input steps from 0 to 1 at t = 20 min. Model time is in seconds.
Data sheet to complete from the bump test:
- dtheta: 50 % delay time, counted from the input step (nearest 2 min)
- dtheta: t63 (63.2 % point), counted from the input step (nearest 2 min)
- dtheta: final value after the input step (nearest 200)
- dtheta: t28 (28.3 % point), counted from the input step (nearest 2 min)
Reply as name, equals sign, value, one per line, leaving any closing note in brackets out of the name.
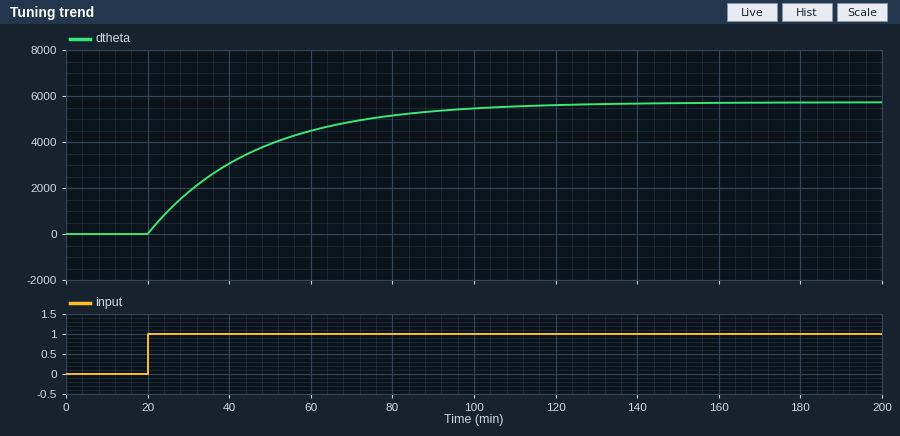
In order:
dtheta: 50 % delay time, counted from the input step = 18 min
dtheta: t63 (63.2 % point), counted from the input step = 26 min
dtheta: final value after the input step = 5800
dtheta: t28 (28.3 % point), counted from the input step = 8 min
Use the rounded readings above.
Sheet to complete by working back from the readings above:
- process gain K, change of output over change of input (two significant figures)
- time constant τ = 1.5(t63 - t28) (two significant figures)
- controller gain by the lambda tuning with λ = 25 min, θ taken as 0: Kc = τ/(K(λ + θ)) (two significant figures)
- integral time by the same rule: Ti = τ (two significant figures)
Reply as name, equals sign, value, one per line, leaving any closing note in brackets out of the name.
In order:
process gain K, change of output over change of input = 5800
time constant τ = 1.5(t63 - t28) = 27 min
controller gain by the lambda tuning with λ = 25 min, θ taken as 0: Kc = τ/(K(λ + θ)) = 0.00019
integral time by the same rule: Ti = τ = 27 min
